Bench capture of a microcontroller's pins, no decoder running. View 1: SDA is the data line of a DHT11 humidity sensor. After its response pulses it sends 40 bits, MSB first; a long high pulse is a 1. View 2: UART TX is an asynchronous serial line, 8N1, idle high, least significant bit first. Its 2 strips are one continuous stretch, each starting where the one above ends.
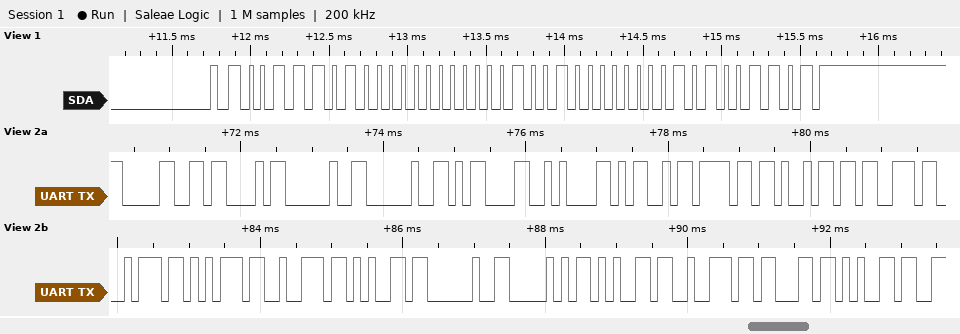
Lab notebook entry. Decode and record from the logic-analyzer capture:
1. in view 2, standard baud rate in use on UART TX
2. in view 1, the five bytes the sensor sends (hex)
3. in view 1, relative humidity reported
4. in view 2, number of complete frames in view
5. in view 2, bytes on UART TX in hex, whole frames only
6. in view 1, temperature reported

9600 baud
3A 00 12 01 4D
58 %
20
30 43 20 20 0D 0A 4D 6F 69 73 74 75 72 65 20 50 65 72 63 65
18.1 °C
